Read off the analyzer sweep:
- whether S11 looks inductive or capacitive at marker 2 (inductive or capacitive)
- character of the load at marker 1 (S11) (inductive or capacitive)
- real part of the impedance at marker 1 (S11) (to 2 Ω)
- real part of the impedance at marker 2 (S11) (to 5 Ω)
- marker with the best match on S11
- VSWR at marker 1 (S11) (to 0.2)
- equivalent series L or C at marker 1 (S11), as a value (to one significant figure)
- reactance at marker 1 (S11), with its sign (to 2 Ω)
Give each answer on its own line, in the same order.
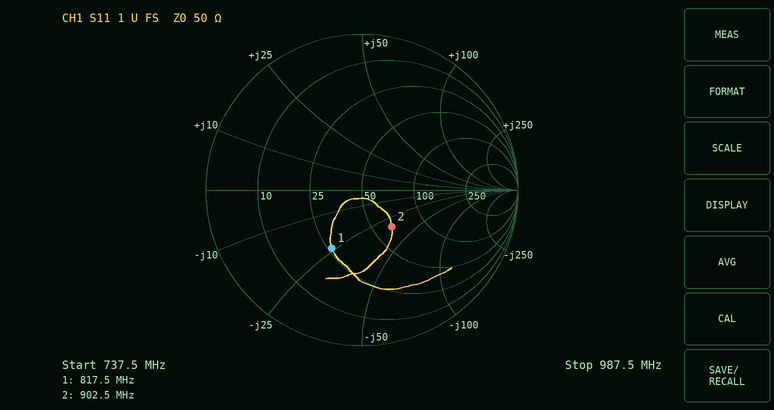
capacitive
capacitive
26 Ω
65 Ω
marker 2
2.4
8 pF
-24 Ω
